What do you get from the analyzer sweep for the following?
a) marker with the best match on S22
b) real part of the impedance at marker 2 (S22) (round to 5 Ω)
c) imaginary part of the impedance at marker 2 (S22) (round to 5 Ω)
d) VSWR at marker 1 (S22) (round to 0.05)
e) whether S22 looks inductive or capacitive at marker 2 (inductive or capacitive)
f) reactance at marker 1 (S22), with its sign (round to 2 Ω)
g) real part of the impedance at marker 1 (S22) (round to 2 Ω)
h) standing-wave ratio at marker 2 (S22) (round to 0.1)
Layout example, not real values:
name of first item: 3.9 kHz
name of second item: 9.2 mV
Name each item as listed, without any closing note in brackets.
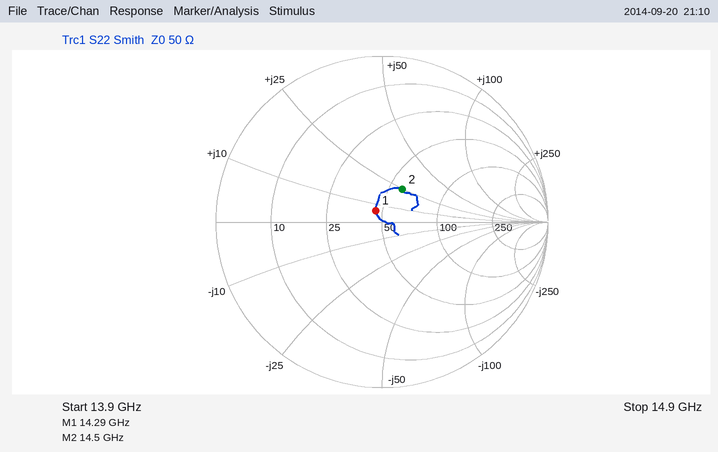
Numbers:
marker with the best match on S22: marker 1
real part of the impedance at marker 2 (S22): 60 Ω
imaginary part of the impedance at marker 2 (S22): +25 Ω
VSWR at marker 1 (S22): 1.15
whether S22 looks inductive or capacitive at marker 2: inductive
reactance at marker 1 (S22), with its sign: +6 Ω
real part of the impedance at marker 1 (S22): 46 Ω
standing-wave ratio at marker 2 (S22): 1.6
